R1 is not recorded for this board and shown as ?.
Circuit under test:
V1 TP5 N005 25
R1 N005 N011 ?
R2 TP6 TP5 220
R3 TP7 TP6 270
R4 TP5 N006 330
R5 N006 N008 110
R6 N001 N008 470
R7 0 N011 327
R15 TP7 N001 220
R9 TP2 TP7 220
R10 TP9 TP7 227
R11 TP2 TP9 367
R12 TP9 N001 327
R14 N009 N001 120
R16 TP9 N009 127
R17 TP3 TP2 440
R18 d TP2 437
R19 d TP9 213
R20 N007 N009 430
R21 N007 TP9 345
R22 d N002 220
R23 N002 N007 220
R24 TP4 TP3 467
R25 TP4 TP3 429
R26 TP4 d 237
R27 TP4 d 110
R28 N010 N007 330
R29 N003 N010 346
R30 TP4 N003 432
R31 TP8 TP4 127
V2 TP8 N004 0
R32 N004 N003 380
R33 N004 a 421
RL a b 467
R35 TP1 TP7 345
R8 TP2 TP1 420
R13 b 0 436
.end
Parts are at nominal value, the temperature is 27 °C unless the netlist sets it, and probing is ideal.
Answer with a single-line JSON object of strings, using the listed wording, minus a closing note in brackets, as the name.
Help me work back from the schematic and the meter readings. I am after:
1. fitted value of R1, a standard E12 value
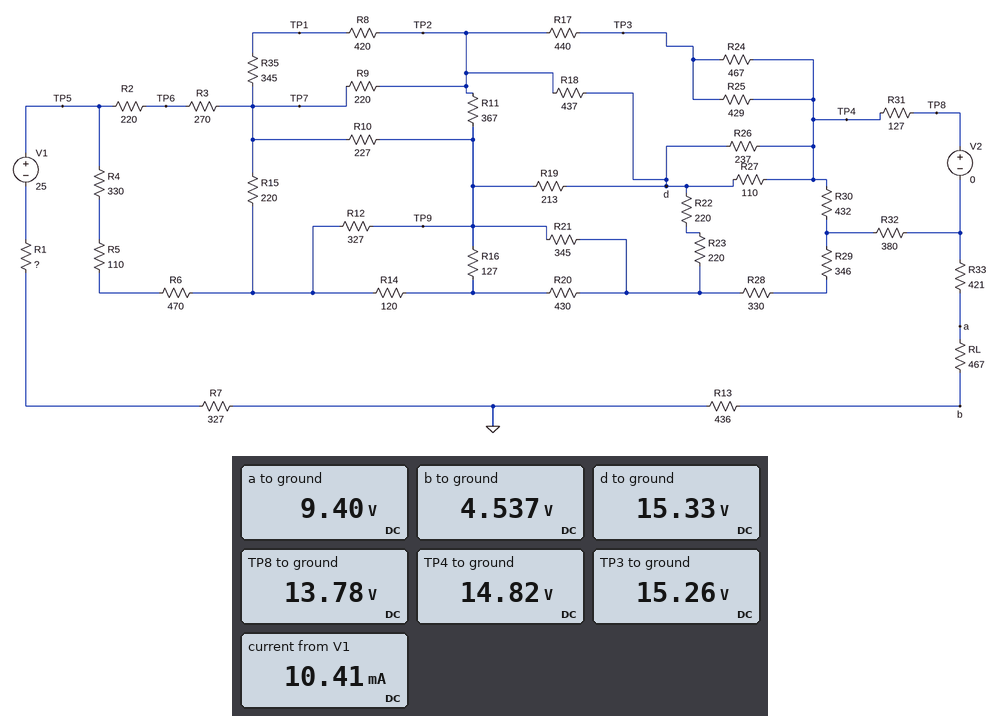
{"fitted value of R1, a standard E12 value": "150 Ω"}
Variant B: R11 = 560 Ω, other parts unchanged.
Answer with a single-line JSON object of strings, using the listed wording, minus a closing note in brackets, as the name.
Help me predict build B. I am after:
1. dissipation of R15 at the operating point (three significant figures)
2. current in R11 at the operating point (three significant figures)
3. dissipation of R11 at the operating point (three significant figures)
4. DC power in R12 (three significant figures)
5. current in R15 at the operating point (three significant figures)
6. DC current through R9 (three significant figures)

{"dissipation of R15 at the operating point": "42.4 µW", "current in R11 at the operating point": "91.6 µA", "dissipation of R11 at the operating point": "4.70 µW", "DC power in R12": "716 µW", "current in R15 at the operating point": "439 µA", "DC current through R9": "2.87 mA"}
